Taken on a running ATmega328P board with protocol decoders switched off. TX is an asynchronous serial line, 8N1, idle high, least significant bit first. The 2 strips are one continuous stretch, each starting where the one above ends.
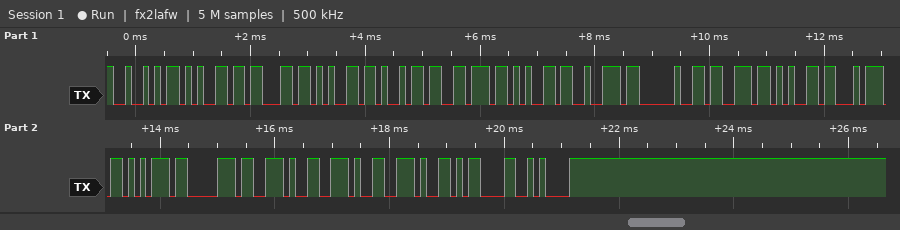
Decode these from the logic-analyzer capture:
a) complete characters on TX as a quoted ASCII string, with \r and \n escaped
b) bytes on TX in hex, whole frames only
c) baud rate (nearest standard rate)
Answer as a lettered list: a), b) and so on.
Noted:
a) "Receiver setup...\r\n"
b) 0x52 0x65 0x63 0x65 0x69 0x76 0x65 0x72 0x20 0x73 0x65 0x74 0x75 0x70 0x2E 0x2E 0x2E 0x0D 0x0A
c) 9600 baud
